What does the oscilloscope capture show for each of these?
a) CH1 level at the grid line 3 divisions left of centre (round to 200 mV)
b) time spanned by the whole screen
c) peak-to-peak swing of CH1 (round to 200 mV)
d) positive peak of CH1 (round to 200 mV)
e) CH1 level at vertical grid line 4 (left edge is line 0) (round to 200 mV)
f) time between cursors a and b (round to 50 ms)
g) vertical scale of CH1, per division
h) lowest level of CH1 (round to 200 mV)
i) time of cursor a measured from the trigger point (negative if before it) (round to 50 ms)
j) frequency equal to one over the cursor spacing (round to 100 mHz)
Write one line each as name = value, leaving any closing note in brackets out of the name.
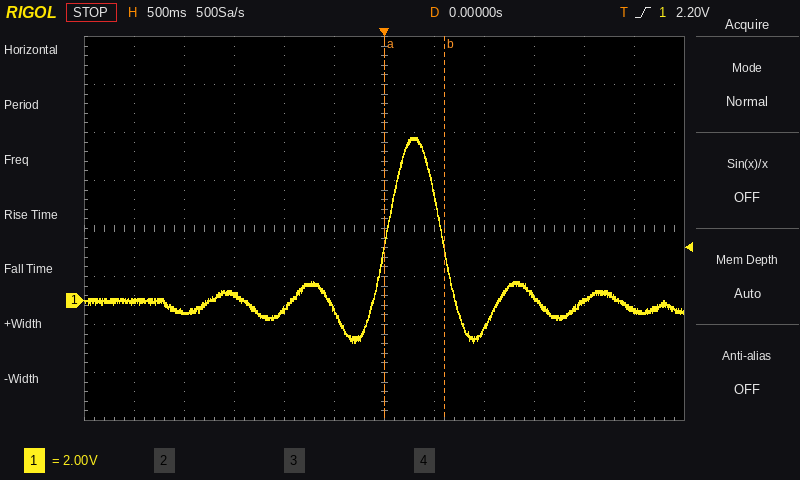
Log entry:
CH1 level at the grid line 3 divisions left of centre = 200 mV
time spanned by the whole screen = 6 s
peak-to-peak swing of CH1 = 8.6 V
positive peak of CH1 = 6.8 V
CH1 level at vertical grid line 4 (left edge is line 0) = -400 mV
time between cursors a and b = 600 ms
vertical scale of CH1, per division = 2 V
lowest level of CH1 = -1.8 V
time of cursor a measured from the trigger point (negative if before it) = 0 ms
frequency equal to one over the cursor spacing = 1.7 Hz
